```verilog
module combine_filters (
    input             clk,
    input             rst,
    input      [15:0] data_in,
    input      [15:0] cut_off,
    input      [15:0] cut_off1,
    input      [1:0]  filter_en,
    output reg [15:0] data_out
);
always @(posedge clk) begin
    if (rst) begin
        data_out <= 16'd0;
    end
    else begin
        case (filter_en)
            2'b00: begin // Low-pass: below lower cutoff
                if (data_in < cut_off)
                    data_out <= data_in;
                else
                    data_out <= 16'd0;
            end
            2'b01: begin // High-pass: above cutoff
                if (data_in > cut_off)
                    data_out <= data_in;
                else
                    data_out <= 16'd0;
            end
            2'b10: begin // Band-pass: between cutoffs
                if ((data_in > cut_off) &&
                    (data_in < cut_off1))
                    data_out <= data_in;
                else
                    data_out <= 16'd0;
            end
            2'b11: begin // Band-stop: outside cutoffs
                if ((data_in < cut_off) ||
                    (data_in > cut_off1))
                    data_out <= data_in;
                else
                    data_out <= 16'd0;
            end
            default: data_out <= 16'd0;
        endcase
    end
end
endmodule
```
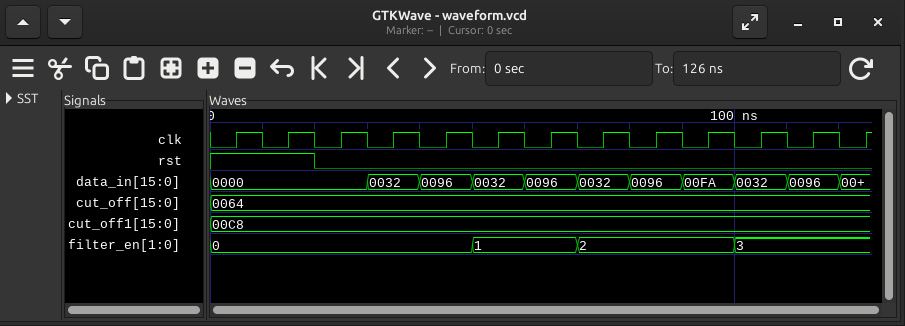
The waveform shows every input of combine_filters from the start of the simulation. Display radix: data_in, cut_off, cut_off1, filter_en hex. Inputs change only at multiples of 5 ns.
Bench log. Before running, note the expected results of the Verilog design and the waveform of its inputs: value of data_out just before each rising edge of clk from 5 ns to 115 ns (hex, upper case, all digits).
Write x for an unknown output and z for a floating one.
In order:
x, 0000, 0000, 0000, 0032, 0000, 0000, 0096, 0000, 0096, 0000, 0032
